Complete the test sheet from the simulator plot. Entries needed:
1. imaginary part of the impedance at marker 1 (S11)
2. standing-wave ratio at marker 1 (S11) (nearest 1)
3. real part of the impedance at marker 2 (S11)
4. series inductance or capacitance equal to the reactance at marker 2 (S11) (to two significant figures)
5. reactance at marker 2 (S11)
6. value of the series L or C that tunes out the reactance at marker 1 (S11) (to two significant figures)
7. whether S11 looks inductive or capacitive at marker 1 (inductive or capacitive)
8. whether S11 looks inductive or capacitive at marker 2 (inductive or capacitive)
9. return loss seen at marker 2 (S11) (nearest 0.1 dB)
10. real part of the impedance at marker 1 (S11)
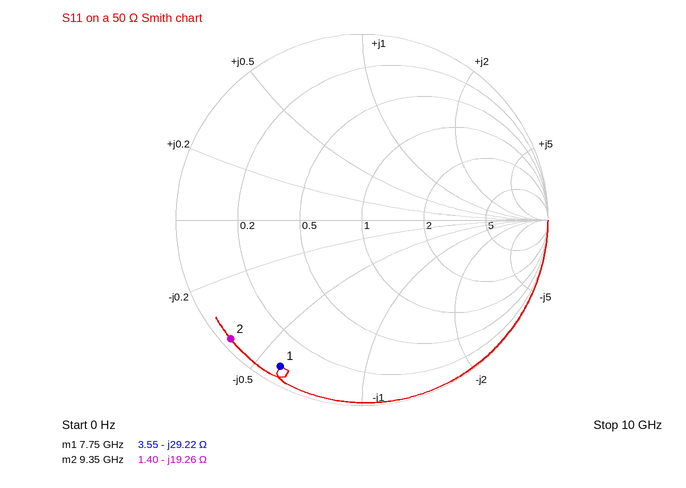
-29.22 Ω
19
1.40 Ω
880 fF
-19.26 Ω
600 pH
capacitive
capacitive
0.4 dB
3.55 Ω
